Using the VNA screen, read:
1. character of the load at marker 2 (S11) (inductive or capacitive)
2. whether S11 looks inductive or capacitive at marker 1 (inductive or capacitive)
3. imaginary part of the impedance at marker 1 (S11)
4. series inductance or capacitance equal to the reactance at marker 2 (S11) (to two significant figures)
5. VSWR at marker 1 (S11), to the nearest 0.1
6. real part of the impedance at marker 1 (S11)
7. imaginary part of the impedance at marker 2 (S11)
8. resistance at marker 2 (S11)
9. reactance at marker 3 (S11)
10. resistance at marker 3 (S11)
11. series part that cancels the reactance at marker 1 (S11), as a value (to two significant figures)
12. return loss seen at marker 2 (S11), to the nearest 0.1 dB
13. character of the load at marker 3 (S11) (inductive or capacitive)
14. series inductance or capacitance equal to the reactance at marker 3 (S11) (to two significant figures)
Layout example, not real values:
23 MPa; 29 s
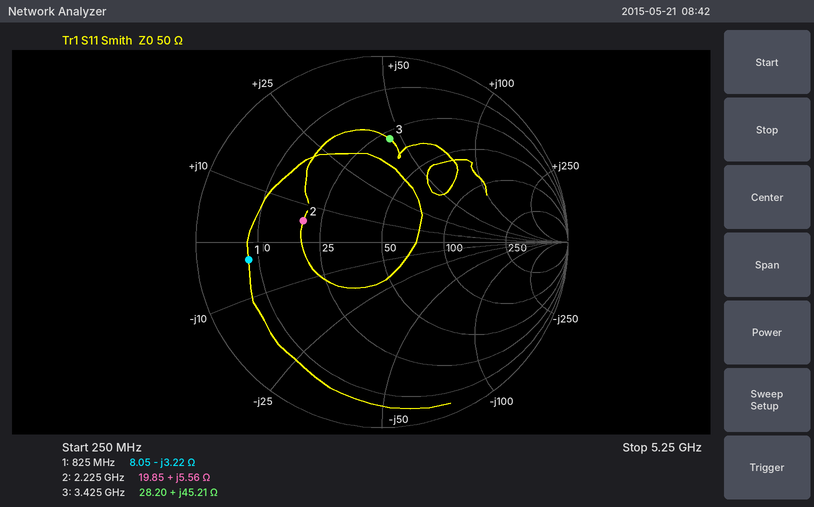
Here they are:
inductive; capacitive; -3.22 Ω; 400 pH; 6.2; 8.05 Ω; +5.56 Ω; 19.85 Ω; +45.21 Ω; 28.20 Ω; 620 pH; 7.2 dB; inductive; 2.1 nH
